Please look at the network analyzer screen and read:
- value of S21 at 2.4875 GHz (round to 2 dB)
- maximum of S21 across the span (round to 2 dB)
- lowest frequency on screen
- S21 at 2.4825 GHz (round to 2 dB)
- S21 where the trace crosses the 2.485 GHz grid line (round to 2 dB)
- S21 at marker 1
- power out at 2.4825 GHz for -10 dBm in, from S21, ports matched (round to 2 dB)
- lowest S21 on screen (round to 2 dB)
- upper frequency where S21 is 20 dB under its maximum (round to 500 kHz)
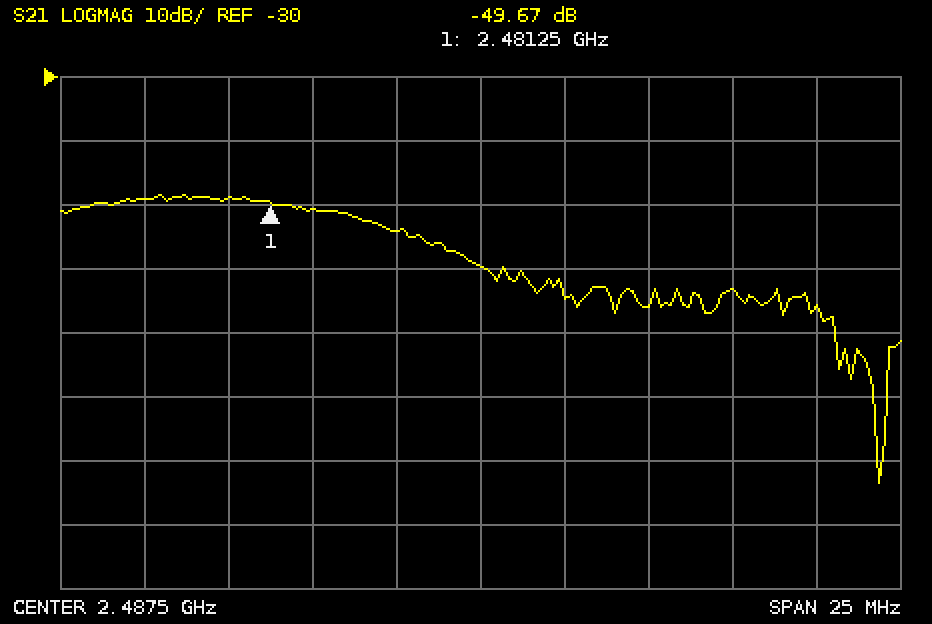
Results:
-60 dB
-48 dB
2.475 GHz
-50 dB
-54 dB
-49.67 dB
-60 dBm
-94 dB
2.4980 GHz
